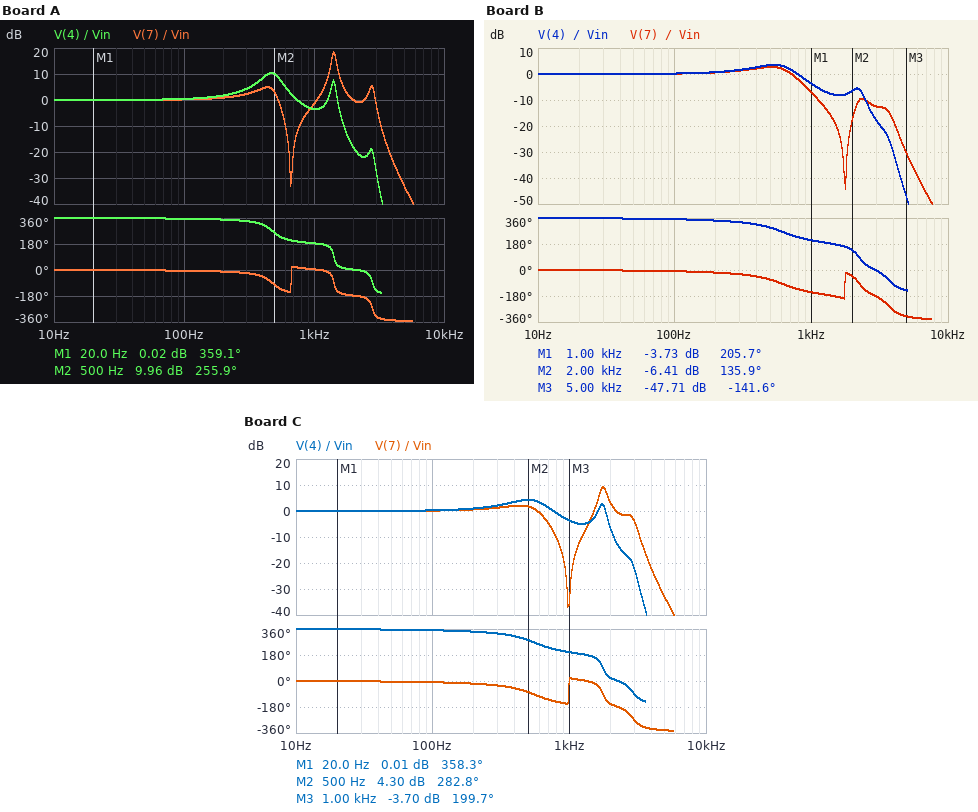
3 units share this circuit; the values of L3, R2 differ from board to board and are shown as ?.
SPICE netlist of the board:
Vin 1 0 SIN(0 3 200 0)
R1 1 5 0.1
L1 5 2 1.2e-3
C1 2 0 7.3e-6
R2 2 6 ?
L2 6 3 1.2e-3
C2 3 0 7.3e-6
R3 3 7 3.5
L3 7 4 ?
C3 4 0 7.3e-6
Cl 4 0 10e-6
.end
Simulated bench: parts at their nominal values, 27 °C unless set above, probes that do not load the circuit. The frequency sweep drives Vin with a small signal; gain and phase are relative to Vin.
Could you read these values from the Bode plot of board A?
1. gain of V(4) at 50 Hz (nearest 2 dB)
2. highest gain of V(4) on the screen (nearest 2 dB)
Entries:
0 dB
10 dB
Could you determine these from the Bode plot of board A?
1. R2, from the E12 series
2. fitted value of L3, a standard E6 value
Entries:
2.7 Ω
3.3 mH
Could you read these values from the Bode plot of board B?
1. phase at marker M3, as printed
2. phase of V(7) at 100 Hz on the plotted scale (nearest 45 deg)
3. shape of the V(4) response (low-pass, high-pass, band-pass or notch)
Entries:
-141.6 deg
0 deg
low-pass
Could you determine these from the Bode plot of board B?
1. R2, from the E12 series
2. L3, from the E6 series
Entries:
6.8 Ω
470 µH
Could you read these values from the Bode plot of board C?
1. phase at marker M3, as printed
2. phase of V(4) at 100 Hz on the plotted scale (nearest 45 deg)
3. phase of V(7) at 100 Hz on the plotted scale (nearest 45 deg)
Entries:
199.7 deg
360 deg
0 deg
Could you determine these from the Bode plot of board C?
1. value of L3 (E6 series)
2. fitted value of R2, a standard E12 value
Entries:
1.5 mH
6.8 Ω
